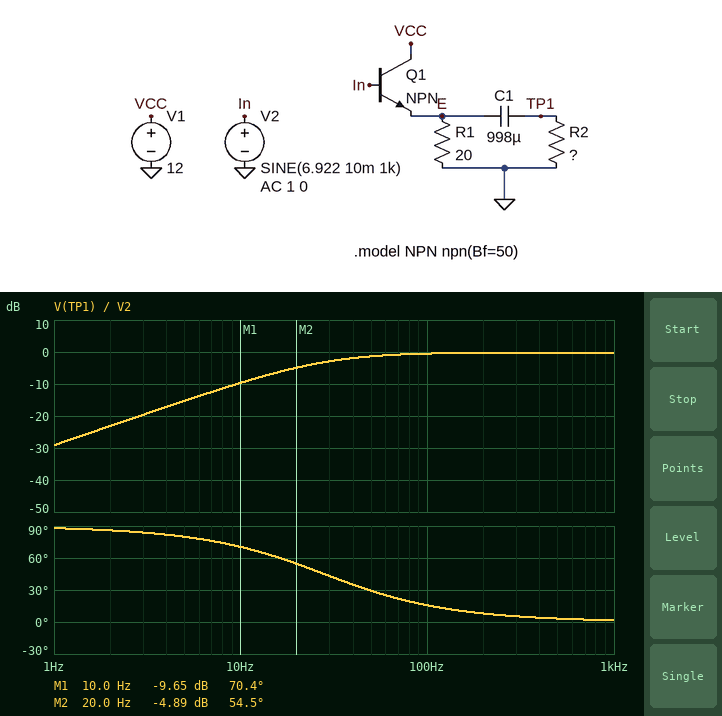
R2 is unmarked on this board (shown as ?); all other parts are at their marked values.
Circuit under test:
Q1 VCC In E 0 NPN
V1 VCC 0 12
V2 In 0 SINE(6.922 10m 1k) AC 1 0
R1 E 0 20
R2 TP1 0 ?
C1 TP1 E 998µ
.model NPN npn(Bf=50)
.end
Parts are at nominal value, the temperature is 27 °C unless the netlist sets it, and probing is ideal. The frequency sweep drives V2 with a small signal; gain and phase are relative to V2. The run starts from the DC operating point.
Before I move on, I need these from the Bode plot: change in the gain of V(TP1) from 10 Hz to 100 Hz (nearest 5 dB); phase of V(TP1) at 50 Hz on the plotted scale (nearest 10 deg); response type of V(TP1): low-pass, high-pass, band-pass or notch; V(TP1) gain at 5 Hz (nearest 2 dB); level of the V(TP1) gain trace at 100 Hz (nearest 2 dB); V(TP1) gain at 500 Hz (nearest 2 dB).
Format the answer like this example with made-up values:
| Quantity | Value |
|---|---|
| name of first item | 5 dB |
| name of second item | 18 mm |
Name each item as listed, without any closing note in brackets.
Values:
| Quantity | Value |
|---|---|
| change in the gain of V(TP1) from 10 Hz to 100 Hz | 10 dB |
| phase of V(TP1) at 50 Hz on the plotted scale | 30 deg |
| response type of V(TP1): low-pass, high-pass, band-pass or notch | high-pass |
| V(TP1) gain at 5 Hz | -16 dB |
| level of the V(TP1) gain trace at 100 Hz | 0 dB |
| V(TP1) gain at 500 Hz | 0 dB |
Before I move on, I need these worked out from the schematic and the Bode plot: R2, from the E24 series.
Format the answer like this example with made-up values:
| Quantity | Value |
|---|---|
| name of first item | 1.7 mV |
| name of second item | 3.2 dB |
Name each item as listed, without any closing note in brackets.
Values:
| Quantity | Value |
|---|---|
| R2, from the E24 series | 5.6 Ω |
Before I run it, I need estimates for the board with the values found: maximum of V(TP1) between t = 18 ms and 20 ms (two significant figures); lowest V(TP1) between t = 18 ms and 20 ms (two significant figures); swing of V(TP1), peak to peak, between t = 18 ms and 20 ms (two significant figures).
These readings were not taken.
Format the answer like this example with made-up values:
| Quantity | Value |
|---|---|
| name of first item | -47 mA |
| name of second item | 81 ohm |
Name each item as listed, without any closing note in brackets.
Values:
| Quantity | Value |
|---|---|
| maximum of V(TP1) between t = 18 ms and 20 ms | 9.8 mV |
| lowest V(TP1) between t = 18 ms and 20 ms | -9.8 mV |
| swing of V(TP1), peak to peak, between t = 18 ms and 20 ms | 20 mV |
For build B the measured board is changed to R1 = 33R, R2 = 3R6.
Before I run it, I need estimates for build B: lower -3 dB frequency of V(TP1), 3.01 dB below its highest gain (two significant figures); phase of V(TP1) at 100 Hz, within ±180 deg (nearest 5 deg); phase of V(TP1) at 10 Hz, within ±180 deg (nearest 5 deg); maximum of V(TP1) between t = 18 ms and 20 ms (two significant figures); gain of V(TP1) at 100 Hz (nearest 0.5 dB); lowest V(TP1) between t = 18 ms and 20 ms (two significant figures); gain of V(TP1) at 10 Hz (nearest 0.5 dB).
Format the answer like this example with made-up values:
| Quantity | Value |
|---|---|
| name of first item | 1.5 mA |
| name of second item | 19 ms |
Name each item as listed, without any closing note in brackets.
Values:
| Quantity | Value |
|---|---|
| lower -3 dB frequency of V(TP1), 3.01 dB below its highest gain | 43 Hz |
| phase of V(TP1) at 100 Hz, within ±180 deg | 25 deg |
| phase of V(TP1) at 10 Hz, within ±180 deg | 75 deg |
| maximum of V(TP1) between t = 18 ms and 20 ms | 9.6 mV |
| gain of V(TP1) at 100 Hz | -1.0 dB |
| lowest V(TP1) between t = 18 ms and 20 ms | -9.6 mV |
| gain of V(TP1) at 10 Hz | -13.0 dB |
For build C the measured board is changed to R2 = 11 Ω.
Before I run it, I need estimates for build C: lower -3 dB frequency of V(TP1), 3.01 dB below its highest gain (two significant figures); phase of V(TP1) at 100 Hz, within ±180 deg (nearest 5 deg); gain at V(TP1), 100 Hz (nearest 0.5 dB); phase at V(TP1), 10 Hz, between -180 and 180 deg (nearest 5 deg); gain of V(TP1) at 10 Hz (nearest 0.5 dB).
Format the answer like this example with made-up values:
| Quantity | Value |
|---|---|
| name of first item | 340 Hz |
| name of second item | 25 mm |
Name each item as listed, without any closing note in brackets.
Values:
| Quantity | Value |
|---|---|
| lower -3 dB frequency of V(TP1), 3.01 dB below its highest gain | 14 Hz |
| phase of V(TP1) at 100 Hz, within ±180 deg | 10 deg |
| gain at V(TP1), 100 Hz | 0 dB |
| phase at V(TP1), 10 Hz, between -180 and 180 deg | 55 deg |
| gain of V(TP1) at 10 Hz | -5.0 dB |
